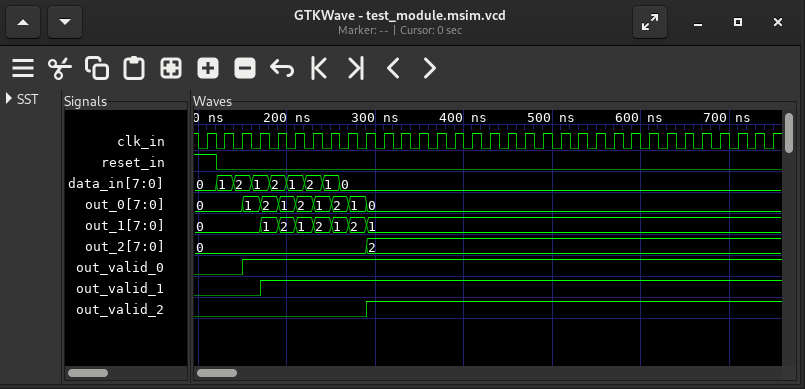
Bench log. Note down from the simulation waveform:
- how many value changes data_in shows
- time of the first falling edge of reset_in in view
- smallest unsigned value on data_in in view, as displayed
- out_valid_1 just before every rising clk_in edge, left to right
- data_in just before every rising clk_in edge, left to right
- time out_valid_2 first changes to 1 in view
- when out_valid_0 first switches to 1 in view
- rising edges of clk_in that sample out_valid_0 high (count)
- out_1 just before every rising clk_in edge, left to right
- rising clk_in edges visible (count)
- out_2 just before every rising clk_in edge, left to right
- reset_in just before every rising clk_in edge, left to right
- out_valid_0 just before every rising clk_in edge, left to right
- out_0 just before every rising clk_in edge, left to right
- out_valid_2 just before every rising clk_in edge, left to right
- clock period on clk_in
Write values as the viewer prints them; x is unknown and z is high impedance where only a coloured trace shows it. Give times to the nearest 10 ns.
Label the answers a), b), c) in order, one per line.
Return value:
a) 8
b) 120 ns
c) 0
d) 0 0 0 0 1 1 1 1 1 1 1 1 1 1 1 1 1 1 1 1 1 1 1 1 1 1 1 1 1 1 1 1 1
e) 0, 1, 2, 1, 2, 1, 2, 1, 0, 0, 0, 0, 0, 0, 0, 0, 0, 0, 0, 0, 0, 0, 0, 0, 0, 0, 0, 0, 0, 0, 0, 0, 0
f) 290 ns
g) 150 ns
h) 30
i) 0, 0, 0, 0, 1, 2, 1, 2, 1, 2, 1, 1, 1, 1, 1, 1, 1, 1, 1, 1, 1, 1, 1, 1, 1, 1, 1, 1, 1, 1, 1, 1, 1
j) 33
k) 0, 0, 0, 0, 0, 0, 0, 0, 0, 0, 2, 2, 2, 2, 2, 2, 2, 2, 2, 2, 2, 2, 2, 2, 2, 2, 2, 2, 2, 2, 2, 2, 2
l) 1 0 0 0 0 0 0 0 0 0 0 0 0 0 0 0 0 0 0 0 0 0 0 0 0 0 0 0 0 0 0 0 0
m) 0 0 0 1 1 1 1 1 1 1 1 1 1 1 1 1 1 1 1 1 1 1 1 1 1 1 1 1 1 1 1 1 1
n) 0, 0, 0, 1, 2, 1, 2, 1, 2, 1, 0, 0, 0, 0, 0, 0, 0, 0, 0, 0, 0, 0, 0, 0, 0, 0, 0, 0, 0, 0, 0, 0, 0
o) 0 0 0 0 0 0 0 0 0 0 1 1 1 1 1 1 1 1 1 1 1 1 1 1 1 1 1 1 1 1 1 1 1
p) 20 ns
